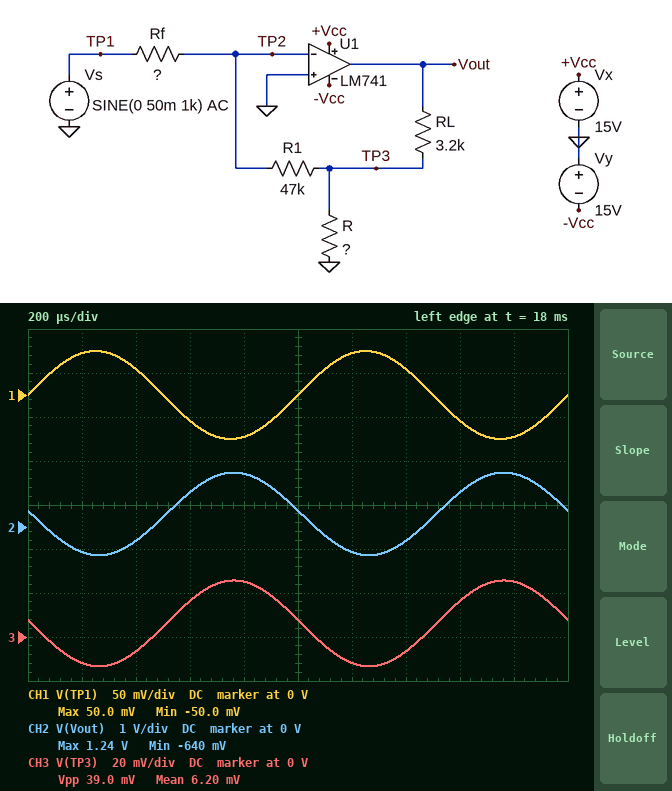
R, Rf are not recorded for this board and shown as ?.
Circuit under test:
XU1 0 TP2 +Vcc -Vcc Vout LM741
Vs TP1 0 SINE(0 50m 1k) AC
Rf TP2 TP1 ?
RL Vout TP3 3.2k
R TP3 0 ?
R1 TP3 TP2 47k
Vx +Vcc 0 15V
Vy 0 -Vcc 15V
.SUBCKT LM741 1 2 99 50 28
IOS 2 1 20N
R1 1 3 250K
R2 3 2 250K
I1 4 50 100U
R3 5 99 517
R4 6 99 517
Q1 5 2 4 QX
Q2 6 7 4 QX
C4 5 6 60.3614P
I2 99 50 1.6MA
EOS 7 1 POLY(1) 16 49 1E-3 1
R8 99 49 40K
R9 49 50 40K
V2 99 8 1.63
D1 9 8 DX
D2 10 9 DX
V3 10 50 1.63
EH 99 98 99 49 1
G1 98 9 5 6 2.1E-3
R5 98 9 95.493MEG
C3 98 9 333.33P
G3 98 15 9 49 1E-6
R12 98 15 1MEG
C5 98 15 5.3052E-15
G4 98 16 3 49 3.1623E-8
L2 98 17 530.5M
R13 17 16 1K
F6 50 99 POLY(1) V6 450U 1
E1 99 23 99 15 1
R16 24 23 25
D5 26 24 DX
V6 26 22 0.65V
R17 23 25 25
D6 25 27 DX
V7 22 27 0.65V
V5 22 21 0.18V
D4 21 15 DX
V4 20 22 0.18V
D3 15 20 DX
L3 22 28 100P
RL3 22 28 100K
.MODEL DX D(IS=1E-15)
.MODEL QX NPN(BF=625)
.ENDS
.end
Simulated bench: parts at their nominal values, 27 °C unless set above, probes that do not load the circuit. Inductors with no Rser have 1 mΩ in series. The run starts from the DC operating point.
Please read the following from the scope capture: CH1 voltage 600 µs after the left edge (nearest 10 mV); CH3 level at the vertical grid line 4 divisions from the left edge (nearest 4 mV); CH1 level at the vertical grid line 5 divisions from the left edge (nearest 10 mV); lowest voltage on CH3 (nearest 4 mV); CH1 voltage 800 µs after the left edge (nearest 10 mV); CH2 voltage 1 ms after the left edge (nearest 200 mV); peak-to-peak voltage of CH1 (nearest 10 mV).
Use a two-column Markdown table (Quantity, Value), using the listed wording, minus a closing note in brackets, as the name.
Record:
| Quantity | Value |
|---|---|
| CH1 voltage 600 µs after the left edge | -30 mV |
| CH3 level at the vertical grid line 4 divisions from the left edge | 24 mV |
| CH1 level at the vertical grid line 5 divisions from the left edge | 0 V |
| lowest voltage on CH3 | -12 mV |
| CH1 voltage 800 µs after the left edge | -50 mV |
| CH2 voltage 1 ms after the left edge | 400 mV |
| peak-to-peak voltage of CH1 | 100 mV |
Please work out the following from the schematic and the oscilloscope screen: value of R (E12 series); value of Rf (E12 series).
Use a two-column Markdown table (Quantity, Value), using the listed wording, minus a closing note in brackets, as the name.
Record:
| Quantity | Value |
|---|---|
| value of R | 68 Ω |
| value of Rf | 120 kΩ |
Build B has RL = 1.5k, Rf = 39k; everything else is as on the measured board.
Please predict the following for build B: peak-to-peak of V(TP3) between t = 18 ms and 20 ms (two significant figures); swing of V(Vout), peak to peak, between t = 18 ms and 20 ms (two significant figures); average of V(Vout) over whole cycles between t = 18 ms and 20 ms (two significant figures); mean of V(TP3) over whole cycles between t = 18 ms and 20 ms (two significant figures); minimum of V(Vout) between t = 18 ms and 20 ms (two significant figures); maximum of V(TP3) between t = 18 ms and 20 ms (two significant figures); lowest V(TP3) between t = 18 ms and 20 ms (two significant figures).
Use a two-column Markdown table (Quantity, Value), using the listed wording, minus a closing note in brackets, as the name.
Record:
| Quantity | Value |
|---|---|
| peak-to-peak of V(TP3) between t = 18 ms and 20 ms | 120 mV |
| swing of V(Vout), peak to peak, between t = 18 ms and 20 ms | 2.8 V |
| average of V(Vout) over whole cycles between t = 18 ms and 20 ms | 160 mV |
| mean of V(TP3) over whole cycles between t = 18 ms and 20 ms | 7.0 mV |
| minimum of V(Vout) between t = 18 ms and 20 ms | -1.2 V |
| maximum of V(TP3) between t = 18 ms and 20 ms | 67 mV |
| lowest V(TP3) between t = 18 ms and 20 ms | -53 mV |
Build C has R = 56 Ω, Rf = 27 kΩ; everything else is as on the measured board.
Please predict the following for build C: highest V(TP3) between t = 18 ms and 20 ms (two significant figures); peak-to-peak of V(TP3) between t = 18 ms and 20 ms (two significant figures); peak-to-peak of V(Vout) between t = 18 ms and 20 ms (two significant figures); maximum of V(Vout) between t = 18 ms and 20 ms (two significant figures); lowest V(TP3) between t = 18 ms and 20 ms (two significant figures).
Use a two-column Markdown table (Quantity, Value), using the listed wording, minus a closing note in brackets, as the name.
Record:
| Quantity | Value |
|---|---|
| highest V(TP3) between t = 18 ms and 20 ms | 93 mV |
| peak-to-peak of V(TP3) between t = 18 ms and 20 ms | 170 mV |
| peak-to-peak of V(Vout) between t = 18 ms and 20 ms | 10 V |
| maximum of V(Vout) between t = 18 ms and 20 ms | 5.4 V |
| lowest V(TP3) between t = 18 ms and 20 ms | -78 mV |
